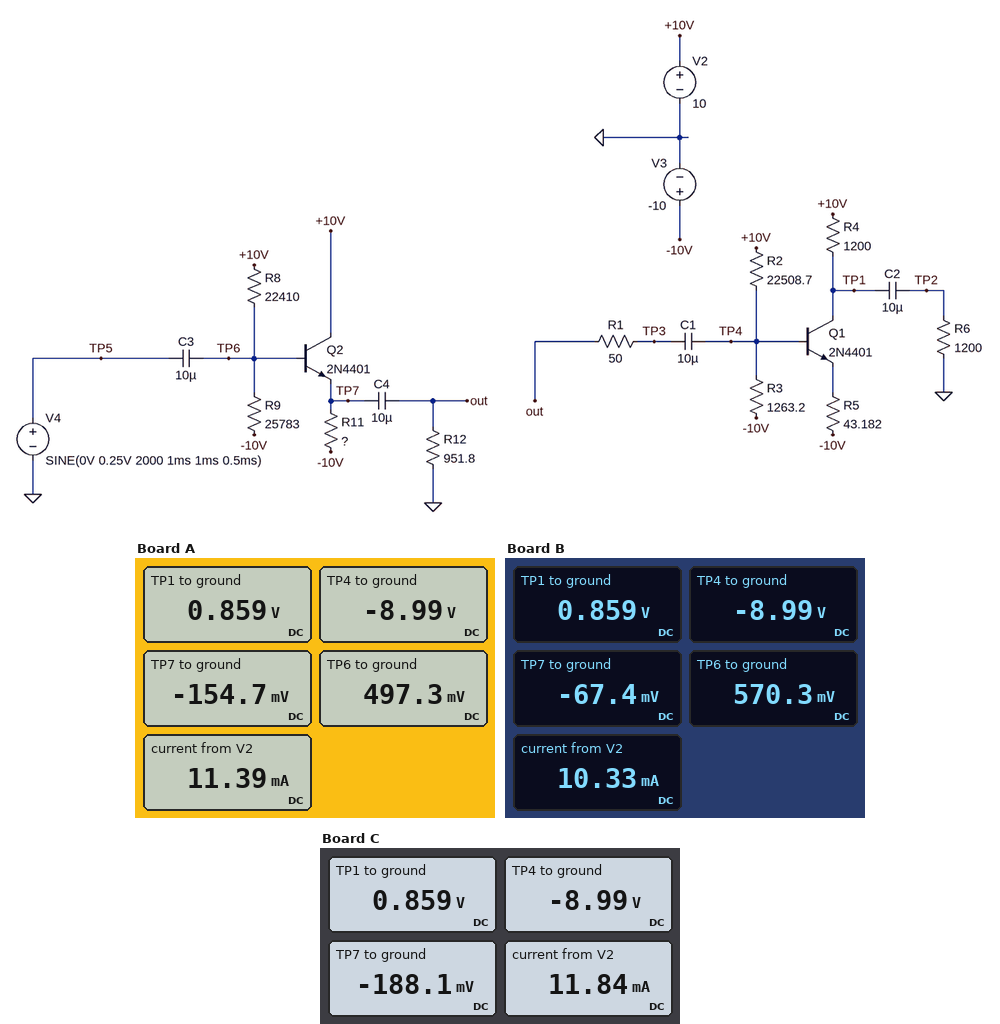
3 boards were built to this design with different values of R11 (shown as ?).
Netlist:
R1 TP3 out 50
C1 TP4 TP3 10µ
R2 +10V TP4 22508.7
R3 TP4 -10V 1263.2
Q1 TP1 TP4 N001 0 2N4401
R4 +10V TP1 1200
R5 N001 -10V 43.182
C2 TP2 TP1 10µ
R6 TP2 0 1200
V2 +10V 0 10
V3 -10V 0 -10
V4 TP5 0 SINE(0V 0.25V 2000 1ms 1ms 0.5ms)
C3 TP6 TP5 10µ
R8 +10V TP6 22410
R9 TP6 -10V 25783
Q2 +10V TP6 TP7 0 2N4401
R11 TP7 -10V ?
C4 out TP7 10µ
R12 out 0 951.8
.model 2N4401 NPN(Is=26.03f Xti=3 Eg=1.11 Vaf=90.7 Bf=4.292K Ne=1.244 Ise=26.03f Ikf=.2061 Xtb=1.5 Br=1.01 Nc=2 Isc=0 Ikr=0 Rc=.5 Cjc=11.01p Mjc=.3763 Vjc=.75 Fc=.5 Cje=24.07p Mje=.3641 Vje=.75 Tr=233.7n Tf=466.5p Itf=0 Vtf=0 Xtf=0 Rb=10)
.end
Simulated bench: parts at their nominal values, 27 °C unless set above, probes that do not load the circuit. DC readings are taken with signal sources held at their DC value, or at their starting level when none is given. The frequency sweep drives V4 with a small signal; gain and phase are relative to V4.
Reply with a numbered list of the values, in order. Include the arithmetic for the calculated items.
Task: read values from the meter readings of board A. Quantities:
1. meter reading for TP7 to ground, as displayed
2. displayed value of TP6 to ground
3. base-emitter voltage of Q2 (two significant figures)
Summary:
1. -154.7 mV
2. 497.3 mV
3. 497.3 mV - (-154.7 mV) = 650 mV
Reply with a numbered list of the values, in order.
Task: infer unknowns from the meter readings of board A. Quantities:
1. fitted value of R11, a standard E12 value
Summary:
1. 3.9 kΩ
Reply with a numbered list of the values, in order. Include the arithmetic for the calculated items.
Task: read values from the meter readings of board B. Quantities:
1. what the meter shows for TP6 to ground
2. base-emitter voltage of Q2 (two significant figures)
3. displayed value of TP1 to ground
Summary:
1. 570.3 mV
2. 570.3 mV - (-67.4 mV) = 640 mV
3. 0.859 V
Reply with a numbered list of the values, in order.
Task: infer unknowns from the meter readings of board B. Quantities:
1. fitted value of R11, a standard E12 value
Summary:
1. 6.8 kΩ
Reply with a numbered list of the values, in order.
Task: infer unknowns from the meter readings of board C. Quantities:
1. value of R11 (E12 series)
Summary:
1. 3.3 kΩ
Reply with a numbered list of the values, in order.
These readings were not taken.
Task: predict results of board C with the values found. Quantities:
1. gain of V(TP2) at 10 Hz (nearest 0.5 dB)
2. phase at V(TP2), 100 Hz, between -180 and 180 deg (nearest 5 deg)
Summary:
1. 6.5 dB
2. -150 deg
